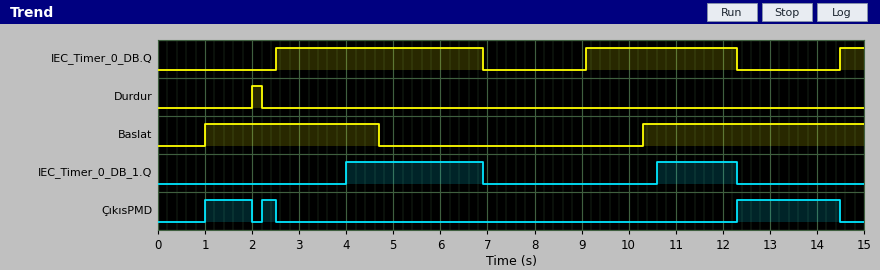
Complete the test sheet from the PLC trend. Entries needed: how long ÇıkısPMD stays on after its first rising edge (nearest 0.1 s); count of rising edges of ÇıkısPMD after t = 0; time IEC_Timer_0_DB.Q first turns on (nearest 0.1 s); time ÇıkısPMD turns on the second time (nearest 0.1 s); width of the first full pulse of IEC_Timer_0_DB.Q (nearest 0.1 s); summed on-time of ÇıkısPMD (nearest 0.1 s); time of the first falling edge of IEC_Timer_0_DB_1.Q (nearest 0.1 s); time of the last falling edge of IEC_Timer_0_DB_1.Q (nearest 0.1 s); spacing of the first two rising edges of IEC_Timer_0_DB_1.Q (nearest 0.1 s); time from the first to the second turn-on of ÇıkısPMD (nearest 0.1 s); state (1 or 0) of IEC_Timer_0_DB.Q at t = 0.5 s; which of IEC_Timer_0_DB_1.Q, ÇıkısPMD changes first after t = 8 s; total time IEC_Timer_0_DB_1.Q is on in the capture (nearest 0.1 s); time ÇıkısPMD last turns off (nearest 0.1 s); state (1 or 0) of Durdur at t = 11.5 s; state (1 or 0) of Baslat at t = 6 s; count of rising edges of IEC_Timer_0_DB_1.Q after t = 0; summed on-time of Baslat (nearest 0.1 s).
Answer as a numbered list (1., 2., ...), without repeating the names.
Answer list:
1. 1.0 s
2. 3
3. 2.5 s
4. 2.2 s
5. 4.4 s
6. 3.5 s
7. 6.9 s
8. 12.3 s
9. 6.6 s
10. 1.2 s
11. 0
12. IEC_Timer_0_DB_1.Q
13. 4.6 s
14. 14.5 s
15. 0
16. 0
17. 2
18. 8.4 s
